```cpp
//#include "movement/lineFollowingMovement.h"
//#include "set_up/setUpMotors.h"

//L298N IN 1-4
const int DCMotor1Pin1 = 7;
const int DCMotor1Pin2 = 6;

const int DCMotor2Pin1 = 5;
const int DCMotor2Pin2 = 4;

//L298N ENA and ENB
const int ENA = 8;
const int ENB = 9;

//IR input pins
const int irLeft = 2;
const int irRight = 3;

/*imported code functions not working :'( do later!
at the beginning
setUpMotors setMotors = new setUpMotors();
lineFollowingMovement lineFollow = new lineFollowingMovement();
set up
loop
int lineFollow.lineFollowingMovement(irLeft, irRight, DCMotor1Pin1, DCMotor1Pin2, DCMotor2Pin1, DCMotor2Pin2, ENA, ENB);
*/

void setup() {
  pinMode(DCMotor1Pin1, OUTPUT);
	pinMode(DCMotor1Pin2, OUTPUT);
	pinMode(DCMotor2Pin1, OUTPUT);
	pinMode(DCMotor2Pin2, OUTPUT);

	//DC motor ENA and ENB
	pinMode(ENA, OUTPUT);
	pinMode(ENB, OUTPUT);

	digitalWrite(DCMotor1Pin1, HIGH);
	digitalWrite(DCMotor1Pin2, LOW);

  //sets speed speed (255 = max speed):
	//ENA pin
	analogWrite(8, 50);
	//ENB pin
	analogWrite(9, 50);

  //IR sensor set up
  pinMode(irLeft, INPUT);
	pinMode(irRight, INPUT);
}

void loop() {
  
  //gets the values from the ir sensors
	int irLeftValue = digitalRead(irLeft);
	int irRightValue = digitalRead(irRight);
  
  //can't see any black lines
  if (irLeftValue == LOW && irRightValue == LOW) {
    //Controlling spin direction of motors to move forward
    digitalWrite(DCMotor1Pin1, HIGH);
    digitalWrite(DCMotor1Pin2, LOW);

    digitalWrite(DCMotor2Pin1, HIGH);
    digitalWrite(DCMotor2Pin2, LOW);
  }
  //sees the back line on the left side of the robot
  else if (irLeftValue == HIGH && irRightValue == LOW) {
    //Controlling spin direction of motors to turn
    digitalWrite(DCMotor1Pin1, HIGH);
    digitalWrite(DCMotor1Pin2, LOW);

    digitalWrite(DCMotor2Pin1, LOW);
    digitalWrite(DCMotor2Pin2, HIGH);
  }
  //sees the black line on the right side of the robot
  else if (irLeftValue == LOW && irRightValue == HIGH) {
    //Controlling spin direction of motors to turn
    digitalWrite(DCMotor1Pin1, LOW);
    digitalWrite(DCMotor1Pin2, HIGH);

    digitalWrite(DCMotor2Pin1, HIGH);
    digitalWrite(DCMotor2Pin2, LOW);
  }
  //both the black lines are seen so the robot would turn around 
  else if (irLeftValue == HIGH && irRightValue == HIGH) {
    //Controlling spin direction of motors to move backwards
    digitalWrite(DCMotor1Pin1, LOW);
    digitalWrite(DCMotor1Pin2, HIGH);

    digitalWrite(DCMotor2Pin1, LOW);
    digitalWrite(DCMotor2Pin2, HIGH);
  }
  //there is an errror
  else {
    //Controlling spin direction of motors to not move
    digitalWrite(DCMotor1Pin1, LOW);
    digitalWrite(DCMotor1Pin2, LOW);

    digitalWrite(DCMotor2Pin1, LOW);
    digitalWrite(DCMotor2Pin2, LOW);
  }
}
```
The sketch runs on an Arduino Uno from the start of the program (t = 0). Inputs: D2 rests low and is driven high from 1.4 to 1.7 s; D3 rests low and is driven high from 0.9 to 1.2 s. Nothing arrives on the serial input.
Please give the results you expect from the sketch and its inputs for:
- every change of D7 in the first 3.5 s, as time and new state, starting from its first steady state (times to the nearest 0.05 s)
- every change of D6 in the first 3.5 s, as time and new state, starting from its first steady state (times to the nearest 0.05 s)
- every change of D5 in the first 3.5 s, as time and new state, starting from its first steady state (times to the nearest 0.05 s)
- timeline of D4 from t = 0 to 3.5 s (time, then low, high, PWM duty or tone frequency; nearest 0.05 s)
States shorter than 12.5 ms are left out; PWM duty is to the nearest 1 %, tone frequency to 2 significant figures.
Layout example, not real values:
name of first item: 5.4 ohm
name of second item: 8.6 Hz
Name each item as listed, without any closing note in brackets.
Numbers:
every change of D7 in the first 3.5 s, as time and new state, starting from its first steady state: 0 s high; 0.9 s low; 1.2 s high
every change of D6 in the first 3.5 s, as time and new state, starting from its first steady state: 0 s low; 0.9 s high; 1.2 s low
every change of D5 in the first 3.5 s, as time and new state, starting from its first steady state: 0 s high; 1.4 s low; 1.7 s high
timeline of D4 from t = 0 to 3.5 s: 0 s low; 1.4 s high; 1.7 s low
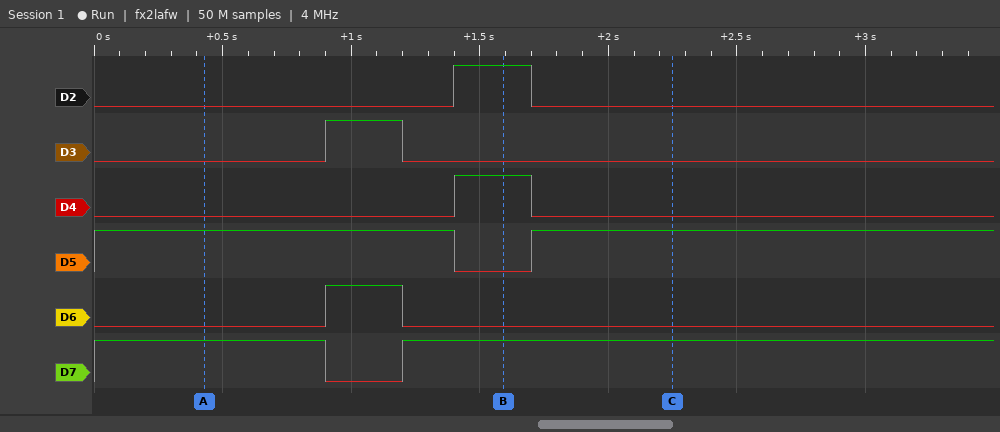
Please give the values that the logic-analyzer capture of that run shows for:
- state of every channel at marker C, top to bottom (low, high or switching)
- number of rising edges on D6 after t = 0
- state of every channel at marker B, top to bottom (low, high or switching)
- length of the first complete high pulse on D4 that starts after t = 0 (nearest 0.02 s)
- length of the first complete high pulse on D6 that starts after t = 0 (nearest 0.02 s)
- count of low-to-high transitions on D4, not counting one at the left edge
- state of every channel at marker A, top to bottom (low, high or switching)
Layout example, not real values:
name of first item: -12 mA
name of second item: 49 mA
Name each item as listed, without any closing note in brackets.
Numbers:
state of every channel at marker C, top to bottom: D2 low, D3 low, D4 low, D5 high, D6 low, D7 high
number of rising edges on D6 after t = 0: 1
state of every channel at marker B, top to bottom: D2 high, D3 low, D4 high, D5 low, D6 low, D7 high
length of the first complete high pulse on D4 that starts after t = 0: 0.30 s
length of the first complete high pulse on D6 that starts after t = 0: 0.30 s
count of low-to-high transitions on D4, not counting one at the left edge: 1
state of every channel at marker A, top to bottom: D2 low, D3 low, D4 low, D5 high, D6 low, D7 high
